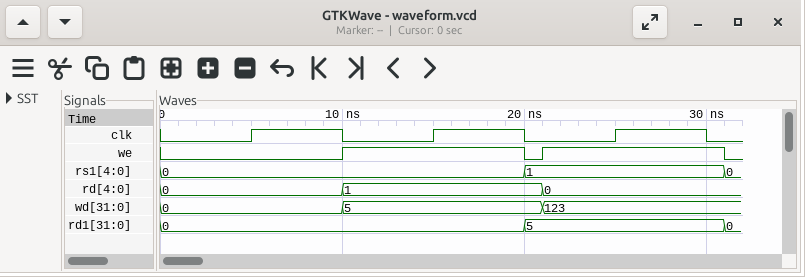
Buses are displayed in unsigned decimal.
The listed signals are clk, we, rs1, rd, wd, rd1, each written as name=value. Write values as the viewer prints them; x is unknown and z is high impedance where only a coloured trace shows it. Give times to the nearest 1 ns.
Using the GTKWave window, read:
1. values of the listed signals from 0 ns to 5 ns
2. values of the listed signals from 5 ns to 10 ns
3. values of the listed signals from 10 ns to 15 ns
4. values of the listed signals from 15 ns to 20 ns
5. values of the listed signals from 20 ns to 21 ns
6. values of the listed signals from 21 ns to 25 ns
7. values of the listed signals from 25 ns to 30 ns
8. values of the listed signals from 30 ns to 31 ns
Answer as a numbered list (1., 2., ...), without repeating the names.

1. clk=0, we=0, rs1=0, rd=0, wd=0, rd1=0
2. clk=1, we=0, rs1=0, rd=0, wd=0, rd1=0
3. clk=0, we=1, rs1=0, rd=1, wd=5, rd1=0
4. clk=1, we=1, rs1=0, rd=1, wd=5, rd1=0
5. clk=0, we=0, rs1=1, rd=1, wd=5, rd1=5
6. clk=0, we=1, rs1=1, rd=0, wd=123, rd1=5
7. clk=1, we=1, rs1=1, rd=0, wd=123, rd1=5
8. clk=0, we=1, rs1=1, rd=0, wd=123, rd1=5
